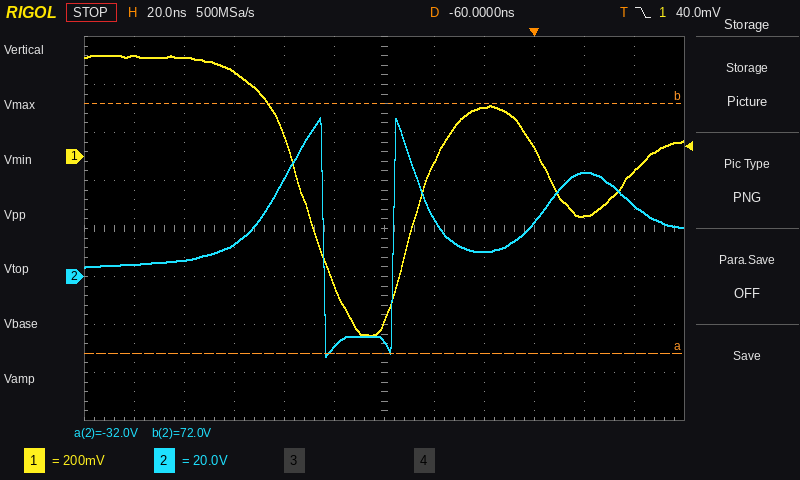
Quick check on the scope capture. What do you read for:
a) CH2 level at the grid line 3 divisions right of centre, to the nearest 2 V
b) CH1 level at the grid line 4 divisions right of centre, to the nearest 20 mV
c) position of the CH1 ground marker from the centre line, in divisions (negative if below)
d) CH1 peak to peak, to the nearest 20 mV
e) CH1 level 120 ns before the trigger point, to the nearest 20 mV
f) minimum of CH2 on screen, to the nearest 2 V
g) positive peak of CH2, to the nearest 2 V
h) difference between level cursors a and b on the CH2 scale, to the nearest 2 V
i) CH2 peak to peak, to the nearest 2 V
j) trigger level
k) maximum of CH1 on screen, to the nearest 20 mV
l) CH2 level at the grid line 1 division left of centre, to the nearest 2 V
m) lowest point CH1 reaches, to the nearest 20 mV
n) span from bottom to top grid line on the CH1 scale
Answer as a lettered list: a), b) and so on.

a) 22 V
b) -240 mV
c) +1.5 div
d) 1.16 V
e) 360 mV
f) -34 V
g) 66 V
h) 104 V
i) 100 V
j) 40.0 mV
k) 420 mV
l) -30 V
m) -740 mV
n) 1.6 V
